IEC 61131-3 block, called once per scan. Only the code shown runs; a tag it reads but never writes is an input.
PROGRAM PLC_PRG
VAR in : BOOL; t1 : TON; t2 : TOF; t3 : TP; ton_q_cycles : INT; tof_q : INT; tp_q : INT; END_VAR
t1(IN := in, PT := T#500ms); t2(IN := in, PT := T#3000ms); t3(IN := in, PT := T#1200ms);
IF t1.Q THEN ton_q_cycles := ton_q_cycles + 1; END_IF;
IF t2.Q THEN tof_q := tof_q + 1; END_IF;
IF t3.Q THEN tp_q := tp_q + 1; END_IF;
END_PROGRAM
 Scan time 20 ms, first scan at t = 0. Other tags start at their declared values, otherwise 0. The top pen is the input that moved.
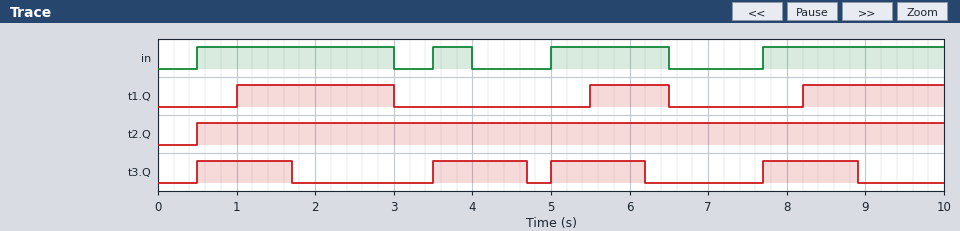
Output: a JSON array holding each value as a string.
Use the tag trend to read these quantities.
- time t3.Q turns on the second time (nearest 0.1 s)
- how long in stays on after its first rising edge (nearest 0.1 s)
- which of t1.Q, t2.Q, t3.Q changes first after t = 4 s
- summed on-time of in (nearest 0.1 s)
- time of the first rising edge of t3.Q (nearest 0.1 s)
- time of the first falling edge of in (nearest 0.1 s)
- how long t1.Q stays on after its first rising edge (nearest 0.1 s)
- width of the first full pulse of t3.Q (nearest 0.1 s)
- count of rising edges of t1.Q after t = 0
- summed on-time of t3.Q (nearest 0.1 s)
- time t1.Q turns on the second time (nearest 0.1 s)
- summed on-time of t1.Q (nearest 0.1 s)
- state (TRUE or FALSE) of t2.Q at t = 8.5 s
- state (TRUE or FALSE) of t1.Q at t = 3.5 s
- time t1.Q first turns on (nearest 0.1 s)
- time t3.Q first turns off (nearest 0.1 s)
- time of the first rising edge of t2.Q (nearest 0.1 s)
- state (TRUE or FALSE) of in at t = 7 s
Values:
["3.5 s", "2.5 s", "t3.Q", "6.8 s", "0.5 s", "3.0 s", "2.0 s", "1.2 s", "3", "4.8 s", "5.5 s", "4.8 s", "TRUE", "FALSE", "1.0 s", "1.7 s", "0.5 s", "FALSE"]
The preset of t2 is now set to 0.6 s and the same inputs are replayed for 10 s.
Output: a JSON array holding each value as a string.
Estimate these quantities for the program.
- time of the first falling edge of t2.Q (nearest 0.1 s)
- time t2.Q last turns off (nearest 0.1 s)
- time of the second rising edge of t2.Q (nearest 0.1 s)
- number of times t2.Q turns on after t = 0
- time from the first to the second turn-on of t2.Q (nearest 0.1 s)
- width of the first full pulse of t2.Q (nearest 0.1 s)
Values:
["4.6 s", "7.1 s", "5.0 s", "3", "4.5 s", "4.1 s"]
